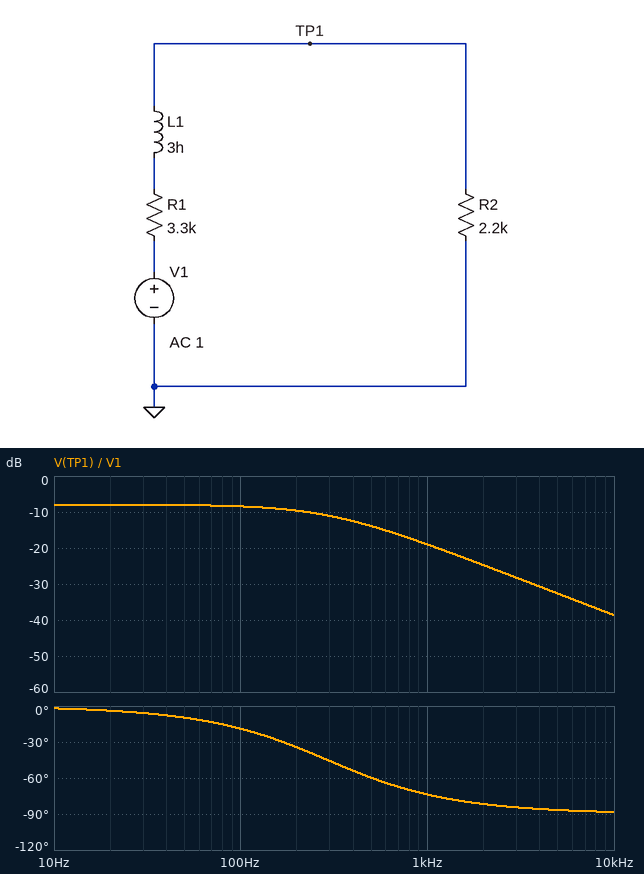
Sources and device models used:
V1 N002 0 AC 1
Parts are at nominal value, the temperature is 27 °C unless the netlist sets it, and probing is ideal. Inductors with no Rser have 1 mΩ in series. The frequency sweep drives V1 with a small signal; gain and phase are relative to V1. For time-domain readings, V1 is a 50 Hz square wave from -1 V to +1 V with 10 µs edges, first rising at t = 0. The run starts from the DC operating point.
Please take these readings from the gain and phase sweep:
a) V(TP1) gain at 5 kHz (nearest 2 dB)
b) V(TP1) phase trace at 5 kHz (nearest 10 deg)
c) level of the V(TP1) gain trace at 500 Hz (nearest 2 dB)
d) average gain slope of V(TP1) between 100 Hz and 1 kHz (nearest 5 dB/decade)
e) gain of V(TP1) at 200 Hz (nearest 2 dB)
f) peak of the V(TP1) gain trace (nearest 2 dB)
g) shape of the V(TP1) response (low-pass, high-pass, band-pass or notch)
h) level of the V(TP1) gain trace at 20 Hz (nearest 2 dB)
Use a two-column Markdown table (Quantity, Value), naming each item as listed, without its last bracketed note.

| Quantity | Value |
|---|---|
| V(TP1) gain at 5 kHz | -32 dB |
| V(TP1) phase trace at 5 kHz | -90 deg |
| level of the V(TP1) gain trace at 500 Hz | -14 dB |
| average gain slope of V(TP1) between 100 Hz and 1 kHz | -10 dB/decade |
| gain of V(TP1) at 200 Hz | -10 dB |
| peak of the V(TP1) gain trace | -8 dB |
| shape of the V(TP1) response | low-pass |
| level of the V(TP1) gain trace at 20 Hz | -8 dB |
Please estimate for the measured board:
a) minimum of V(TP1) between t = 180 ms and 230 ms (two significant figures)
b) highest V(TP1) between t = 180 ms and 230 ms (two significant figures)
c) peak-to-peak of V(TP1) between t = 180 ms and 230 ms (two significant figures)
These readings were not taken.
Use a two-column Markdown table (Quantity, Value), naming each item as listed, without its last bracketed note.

| Quantity | Value |
|---|---|
| minimum of V(TP1) between t = 180 ms and 230 ms | -400 mV |
| highest V(TP1) between t = 180 ms and 230 ms | 400 mV |
| peak-to-peak of V(TP1) between t = 180 ms and 230 ms | 800 mV |
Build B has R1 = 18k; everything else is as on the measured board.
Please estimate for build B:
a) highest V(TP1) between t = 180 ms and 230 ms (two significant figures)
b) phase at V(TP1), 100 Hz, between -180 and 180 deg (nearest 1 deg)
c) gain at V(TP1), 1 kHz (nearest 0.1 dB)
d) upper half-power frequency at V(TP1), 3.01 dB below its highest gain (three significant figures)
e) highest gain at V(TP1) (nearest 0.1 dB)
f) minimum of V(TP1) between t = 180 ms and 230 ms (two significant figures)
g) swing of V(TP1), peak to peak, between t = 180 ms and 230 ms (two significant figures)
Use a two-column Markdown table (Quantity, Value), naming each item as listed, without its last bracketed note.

| Quantity | Value |
|---|---|
| highest V(TP1) between t = 180 ms and 230 ms | 110 mV |
| phase at V(TP1), 100 Hz, between -180 and 180 deg | -5 deg |
| gain at V(TP1), 1 kHz | -22.0 dB |
| upper half-power frequency at V(TP1), 3.01 dB below its highest gain | 1.07 kHz |
| highest gain at V(TP1) | -19.3 dB |
| minimum of V(TP1) between t = 180 ms and 230 ms | -110 mV |
| swing of V(TP1), peak to peak, between t = 180 ms and 230 ms | 220 mV |
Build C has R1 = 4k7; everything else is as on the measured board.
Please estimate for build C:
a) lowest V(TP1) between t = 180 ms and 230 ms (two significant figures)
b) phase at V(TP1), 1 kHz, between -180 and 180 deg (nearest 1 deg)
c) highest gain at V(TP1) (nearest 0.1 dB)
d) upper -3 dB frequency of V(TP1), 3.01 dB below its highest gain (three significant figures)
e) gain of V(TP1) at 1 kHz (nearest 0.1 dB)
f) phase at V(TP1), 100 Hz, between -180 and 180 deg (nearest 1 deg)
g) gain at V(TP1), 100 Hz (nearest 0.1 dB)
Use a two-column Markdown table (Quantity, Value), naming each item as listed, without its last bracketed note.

| Quantity | Value |
|---|---|
| lowest V(TP1) between t = 180 ms and 230 ms | -320 mV |
| phase at V(TP1), 1 kHz, between -180 and 180 deg | -70 deg |
| highest gain at V(TP1) | -9.9 dB |
| upper -3 dB frequency of V(TP1), 3.01 dB below its highest gain | 366 Hz |
| gain of V(TP1) at 1 kHz | -19.2 dB |
| phase at V(TP1), 100 Hz, between -180 and 180 deg | -15 deg |
| gain at V(TP1), 100 Hz | -10.2 dB |
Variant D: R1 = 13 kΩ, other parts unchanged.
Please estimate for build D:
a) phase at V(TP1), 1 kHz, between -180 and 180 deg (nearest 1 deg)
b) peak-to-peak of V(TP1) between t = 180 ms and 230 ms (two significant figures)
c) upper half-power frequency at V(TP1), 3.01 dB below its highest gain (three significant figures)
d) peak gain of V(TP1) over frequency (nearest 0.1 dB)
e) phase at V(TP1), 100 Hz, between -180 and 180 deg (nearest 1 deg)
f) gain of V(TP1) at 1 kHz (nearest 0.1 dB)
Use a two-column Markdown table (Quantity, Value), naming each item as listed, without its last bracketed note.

| Quantity | Value |
|---|---|
| phase at V(TP1), 1 kHz, between -180 and 180 deg | -51 deg |
| peak-to-peak of V(TP1) between t = 180 ms and 230 ms | 290 mV |
| upper half-power frequency at V(TP1), 3.01 dB below its highest gain | 806 Hz |
| peak gain of V(TP1) over frequency | -16.8 dB |
| phase at V(TP1), 100 Hz, between -180 and 180 deg | -7 deg |
| gain of V(TP1) at 1 kHz | -20.8 dB |
